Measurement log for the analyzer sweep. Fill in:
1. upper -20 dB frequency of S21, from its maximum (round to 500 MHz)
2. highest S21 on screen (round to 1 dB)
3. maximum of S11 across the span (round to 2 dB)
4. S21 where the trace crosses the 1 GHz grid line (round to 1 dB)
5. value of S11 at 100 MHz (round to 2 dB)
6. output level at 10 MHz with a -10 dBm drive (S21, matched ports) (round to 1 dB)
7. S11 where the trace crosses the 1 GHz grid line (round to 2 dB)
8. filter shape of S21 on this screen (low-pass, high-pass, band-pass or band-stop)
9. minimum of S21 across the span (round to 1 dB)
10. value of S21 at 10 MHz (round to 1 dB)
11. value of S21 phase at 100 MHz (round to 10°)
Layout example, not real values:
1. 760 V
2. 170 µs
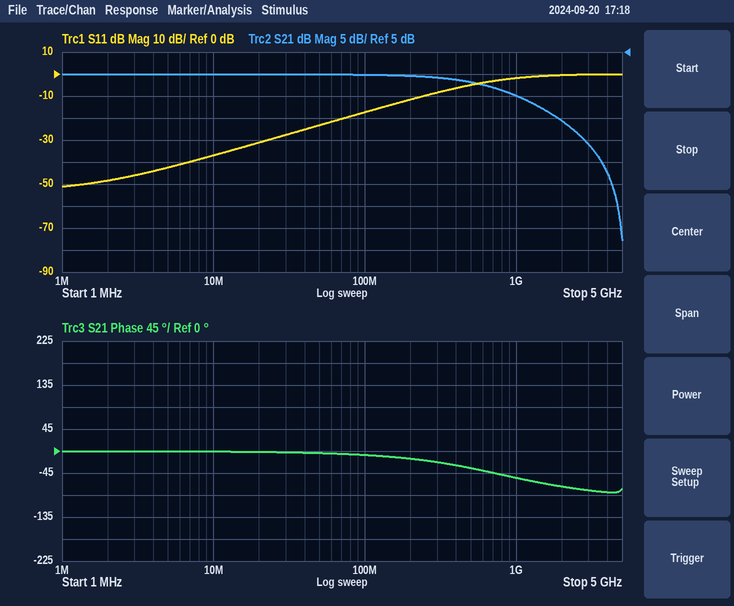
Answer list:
1. 3.5 GHz
2. 0 dB
3. 0 dB
4. -5 dB
5. -18 dB
6. -10 dBm
7. -2 dB
8. low-pass
9. -38 dB
10. 0 dB
11. -10°
